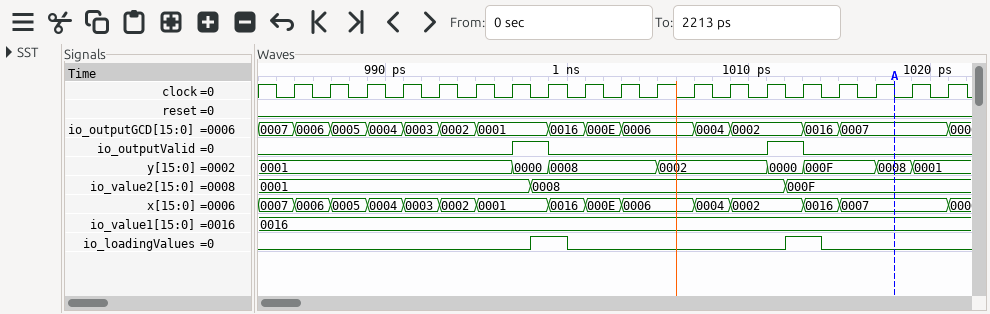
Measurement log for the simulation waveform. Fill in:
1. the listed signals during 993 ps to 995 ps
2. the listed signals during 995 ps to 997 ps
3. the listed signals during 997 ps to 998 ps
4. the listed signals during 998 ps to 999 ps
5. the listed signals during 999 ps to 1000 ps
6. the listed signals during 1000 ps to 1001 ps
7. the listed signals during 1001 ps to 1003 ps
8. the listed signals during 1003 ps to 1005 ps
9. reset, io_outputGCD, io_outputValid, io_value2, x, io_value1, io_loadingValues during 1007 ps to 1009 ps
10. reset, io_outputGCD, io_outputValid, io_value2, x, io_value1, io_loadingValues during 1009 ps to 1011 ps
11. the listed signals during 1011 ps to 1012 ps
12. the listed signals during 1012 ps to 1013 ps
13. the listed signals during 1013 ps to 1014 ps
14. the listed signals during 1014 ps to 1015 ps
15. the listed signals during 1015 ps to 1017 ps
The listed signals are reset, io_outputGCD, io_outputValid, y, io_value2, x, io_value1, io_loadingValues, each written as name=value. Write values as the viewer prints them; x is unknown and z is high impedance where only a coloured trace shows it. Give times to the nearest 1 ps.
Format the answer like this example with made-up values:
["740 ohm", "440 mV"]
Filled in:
["reset=0, io_outputGCD=0002, io_outputValid=0, y=0001, io_value2=0001, x=0002, io_value1=0016, io_loadingValues=0", "reset=0, io_outputGCD=0001, io_outputValid=0, y=0001, io_value2=0001, x=0001, io_value1=0016, io_loadingValues=0", "reset=0, io_outputGCD=0001, io_outputValid=1, y=0000, io_value2=0001, x=0001, io_value1=0016, io_loadingValues=0", "reset=0, io_outputGCD=0001, io_outputValid=1, y=0000, io_value2=0008, x=0001, io_value1=0016, io_loadingValues=1", "reset=0, io_outputGCD=0016, io_outputValid=0, y=0008, io_value2=0008, x=0016, io_value1=0016, io_loadingValues=1", "reset=0, io_outputGCD=0016, io_outputValid=0, y=0008, io_value2=0008, x=0016, io_value1=0016, io_loadingValues=0", "reset=0, io_outputGCD=000E, io_outputValid=0, y=0008, io_value2=0008, x=000E, io_value1=0016, io_loadingValues=0", "reset=0, io_outputGCD=0006, io_outputValid=0, y=0008, io_value2=0008, x=0006, io_value1=0016, io_loadingValues=0", "reset=0, io_outputGCD=0004, io_outputValid=0, io_value2=0008, x=0004, io_value1=0016, io_loadingValues=0", "reset=0, io_outputGCD=0002, io_outputValid=0, io_value2=0008, x=0002, io_value1=0016, io_loadingValues=0", "reset=0, io_outputGCD=0002, io_outputValid=1, y=0000, io_value2=0008, x=0002, io_value1=0016, io_loadingValues=0", "reset=0, io_outputGCD=0002, io_outputValid=1, y=0000, io_value2=000F, x=0002, io_value1=0016, io_loadingValues=1", "reset=0, io_outputGCD=0016, io_outputValid=0, y=000F, io_value2=000F, x=0016, io_value1=0016, io_loadingValues=1", "reset=0, io_outputGCD=0016, io_outputValid=0, y=000F, io_value2=000F, x=0016, io_value1=0016, io_loadingValues=0", "reset=0, io_outputGCD=0007, io_outputValid=0, y=000F, io_value2=000F, x=0007, io_value1=0016, io_loadingValues=0"]
